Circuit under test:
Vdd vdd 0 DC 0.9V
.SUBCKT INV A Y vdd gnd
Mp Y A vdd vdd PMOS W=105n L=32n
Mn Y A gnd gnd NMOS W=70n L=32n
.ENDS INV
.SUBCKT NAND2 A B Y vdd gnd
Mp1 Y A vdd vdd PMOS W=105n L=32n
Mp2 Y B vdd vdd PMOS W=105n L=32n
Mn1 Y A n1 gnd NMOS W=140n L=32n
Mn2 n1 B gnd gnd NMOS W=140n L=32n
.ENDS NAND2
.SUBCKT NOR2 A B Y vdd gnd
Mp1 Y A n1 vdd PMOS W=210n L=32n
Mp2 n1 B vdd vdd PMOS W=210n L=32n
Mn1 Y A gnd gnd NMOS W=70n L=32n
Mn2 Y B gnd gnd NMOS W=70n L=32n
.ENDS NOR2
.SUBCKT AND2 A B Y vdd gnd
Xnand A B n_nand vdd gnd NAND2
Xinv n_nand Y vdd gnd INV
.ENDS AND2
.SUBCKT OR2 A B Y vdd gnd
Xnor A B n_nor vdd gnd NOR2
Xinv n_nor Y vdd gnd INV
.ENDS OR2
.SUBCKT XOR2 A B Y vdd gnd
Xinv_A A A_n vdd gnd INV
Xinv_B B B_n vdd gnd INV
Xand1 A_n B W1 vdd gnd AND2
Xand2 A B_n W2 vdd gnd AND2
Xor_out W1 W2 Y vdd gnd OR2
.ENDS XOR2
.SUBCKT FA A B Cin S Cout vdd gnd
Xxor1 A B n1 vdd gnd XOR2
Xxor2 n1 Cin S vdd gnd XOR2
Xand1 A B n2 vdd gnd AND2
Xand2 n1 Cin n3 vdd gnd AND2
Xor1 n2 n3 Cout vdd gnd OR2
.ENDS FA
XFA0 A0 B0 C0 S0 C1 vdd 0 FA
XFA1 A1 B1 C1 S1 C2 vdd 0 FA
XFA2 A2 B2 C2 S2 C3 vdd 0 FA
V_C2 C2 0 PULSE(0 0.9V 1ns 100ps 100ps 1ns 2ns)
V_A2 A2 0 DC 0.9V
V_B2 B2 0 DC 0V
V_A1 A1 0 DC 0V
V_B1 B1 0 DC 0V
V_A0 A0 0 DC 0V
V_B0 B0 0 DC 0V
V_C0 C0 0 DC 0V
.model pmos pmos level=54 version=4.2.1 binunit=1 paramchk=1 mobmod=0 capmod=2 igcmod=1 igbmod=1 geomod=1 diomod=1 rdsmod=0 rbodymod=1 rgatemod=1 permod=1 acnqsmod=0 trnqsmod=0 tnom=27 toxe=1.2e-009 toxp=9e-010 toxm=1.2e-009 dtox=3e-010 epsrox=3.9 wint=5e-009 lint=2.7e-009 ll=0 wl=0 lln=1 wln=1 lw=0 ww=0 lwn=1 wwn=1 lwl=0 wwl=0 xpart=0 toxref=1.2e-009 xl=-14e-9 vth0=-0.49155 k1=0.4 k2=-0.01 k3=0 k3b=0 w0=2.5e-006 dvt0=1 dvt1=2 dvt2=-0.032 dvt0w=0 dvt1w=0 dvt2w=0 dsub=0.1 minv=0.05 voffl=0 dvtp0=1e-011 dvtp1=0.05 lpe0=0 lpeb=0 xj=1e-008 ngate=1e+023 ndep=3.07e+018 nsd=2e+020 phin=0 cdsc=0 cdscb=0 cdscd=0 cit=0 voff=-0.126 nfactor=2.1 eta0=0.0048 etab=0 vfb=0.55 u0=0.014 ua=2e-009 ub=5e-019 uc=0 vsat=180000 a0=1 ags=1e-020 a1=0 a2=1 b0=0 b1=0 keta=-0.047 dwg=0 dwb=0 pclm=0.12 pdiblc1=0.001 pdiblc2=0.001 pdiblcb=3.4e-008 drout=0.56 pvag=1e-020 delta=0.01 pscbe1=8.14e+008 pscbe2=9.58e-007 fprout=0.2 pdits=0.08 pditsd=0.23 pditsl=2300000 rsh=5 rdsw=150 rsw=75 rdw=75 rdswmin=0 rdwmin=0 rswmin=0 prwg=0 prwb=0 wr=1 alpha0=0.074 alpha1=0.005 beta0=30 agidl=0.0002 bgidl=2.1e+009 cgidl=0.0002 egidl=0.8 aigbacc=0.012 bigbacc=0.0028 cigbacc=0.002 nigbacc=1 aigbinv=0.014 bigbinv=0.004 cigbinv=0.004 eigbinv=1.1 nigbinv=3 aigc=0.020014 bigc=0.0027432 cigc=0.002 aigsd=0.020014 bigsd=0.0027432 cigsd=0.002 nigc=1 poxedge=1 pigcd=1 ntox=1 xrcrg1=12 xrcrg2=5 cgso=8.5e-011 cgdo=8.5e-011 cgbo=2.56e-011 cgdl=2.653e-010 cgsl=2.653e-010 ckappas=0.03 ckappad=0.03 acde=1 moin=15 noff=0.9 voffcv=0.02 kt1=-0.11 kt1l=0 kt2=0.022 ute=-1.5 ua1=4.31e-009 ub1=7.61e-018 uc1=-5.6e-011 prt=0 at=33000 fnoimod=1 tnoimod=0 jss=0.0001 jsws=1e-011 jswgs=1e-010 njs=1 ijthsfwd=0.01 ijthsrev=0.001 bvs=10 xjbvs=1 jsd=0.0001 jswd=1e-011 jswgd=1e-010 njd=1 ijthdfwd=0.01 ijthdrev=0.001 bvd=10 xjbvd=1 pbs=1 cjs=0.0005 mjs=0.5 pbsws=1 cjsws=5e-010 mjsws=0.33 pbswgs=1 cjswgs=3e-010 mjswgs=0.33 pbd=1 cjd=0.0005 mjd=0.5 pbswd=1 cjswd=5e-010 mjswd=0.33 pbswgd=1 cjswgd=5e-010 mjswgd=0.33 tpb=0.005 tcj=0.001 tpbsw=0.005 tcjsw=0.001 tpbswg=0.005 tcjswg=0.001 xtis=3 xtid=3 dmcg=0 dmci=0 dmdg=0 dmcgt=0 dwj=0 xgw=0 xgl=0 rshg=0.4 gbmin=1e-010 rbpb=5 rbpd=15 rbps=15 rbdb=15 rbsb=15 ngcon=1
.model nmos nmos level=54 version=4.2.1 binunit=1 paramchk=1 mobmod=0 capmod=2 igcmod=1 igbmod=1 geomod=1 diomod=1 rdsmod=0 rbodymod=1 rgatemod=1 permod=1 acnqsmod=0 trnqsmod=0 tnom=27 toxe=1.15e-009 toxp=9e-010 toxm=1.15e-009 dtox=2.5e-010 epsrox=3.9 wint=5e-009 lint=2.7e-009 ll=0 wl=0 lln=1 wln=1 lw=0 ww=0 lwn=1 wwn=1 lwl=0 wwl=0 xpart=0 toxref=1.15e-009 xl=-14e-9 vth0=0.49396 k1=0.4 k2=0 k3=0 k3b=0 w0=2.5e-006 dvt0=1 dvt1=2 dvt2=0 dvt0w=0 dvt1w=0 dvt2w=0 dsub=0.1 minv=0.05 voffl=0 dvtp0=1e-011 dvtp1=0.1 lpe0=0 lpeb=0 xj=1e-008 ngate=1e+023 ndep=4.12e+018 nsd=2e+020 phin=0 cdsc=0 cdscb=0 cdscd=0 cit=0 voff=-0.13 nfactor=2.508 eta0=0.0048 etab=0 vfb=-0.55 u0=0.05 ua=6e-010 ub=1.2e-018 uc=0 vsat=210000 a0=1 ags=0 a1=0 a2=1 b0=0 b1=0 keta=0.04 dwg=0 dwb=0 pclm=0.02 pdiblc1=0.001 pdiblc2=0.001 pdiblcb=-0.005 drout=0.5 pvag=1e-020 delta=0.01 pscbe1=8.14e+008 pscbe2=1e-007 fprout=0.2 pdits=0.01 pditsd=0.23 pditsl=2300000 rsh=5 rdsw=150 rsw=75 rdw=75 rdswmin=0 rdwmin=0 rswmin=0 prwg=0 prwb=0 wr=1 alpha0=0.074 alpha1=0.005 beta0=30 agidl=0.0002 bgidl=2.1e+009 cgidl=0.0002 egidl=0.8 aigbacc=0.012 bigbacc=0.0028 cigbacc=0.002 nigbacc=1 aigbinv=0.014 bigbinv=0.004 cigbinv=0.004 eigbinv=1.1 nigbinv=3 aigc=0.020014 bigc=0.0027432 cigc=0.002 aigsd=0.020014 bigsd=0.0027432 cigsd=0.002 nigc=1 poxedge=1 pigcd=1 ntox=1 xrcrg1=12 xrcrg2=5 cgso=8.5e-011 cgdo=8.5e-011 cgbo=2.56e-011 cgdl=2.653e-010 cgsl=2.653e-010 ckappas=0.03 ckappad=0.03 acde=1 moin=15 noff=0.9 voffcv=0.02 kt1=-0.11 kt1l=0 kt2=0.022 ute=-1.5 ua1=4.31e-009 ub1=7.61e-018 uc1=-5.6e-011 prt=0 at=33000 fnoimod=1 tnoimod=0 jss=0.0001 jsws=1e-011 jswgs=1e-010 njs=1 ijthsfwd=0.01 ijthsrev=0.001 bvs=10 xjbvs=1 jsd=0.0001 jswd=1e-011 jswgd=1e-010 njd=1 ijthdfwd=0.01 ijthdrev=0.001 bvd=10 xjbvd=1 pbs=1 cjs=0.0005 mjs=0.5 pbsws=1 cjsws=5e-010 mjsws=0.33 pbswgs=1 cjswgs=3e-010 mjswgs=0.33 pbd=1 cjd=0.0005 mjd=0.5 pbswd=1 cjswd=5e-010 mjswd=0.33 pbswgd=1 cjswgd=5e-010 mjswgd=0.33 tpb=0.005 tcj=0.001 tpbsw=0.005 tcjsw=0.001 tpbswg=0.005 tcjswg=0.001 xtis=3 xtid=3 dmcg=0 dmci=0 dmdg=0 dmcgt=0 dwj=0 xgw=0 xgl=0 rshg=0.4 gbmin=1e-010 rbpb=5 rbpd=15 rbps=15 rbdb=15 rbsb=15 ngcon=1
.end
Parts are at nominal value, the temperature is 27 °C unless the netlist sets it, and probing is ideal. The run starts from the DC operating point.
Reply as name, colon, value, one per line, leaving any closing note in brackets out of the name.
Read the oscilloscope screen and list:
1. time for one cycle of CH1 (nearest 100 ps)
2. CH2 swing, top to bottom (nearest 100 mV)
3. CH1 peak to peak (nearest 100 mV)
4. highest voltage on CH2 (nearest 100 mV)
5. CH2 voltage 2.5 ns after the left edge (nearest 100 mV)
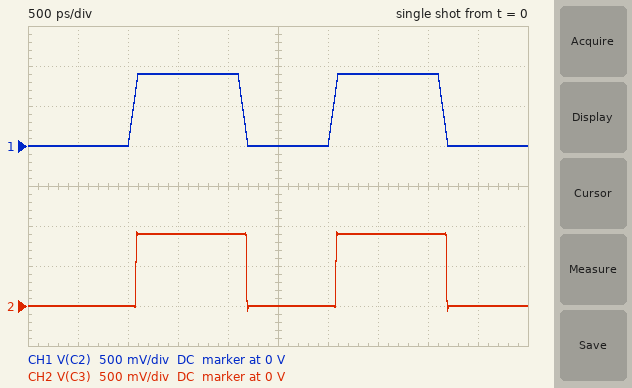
time for one cycle of CH1: 2.0 ns
CH2 swing, top to bottom: 1.0 V
CH1 peak to peak: 900 mV
highest voltage on CH2: 900 mV
CH2 voltage 2.5 ns after the left edge: 0 V
